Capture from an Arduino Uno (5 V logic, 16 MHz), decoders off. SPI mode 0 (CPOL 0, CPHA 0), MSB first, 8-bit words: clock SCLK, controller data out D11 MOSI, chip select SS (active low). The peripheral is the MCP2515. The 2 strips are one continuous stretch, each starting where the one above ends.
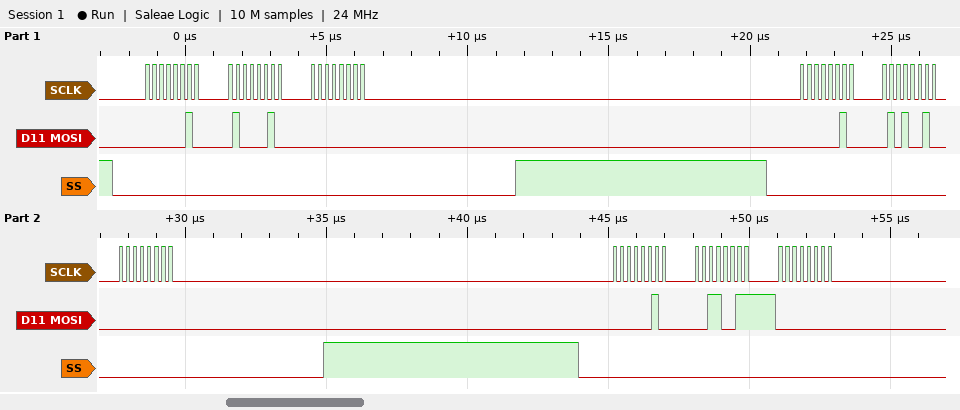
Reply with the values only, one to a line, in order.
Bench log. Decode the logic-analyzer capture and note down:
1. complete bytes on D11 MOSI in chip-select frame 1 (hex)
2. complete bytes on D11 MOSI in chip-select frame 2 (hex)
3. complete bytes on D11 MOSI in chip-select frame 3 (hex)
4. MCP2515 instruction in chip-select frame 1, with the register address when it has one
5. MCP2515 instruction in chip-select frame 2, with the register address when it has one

02 42 00
02 52 00
02 33 00
WRITE 0x42
WRITE 0x52
